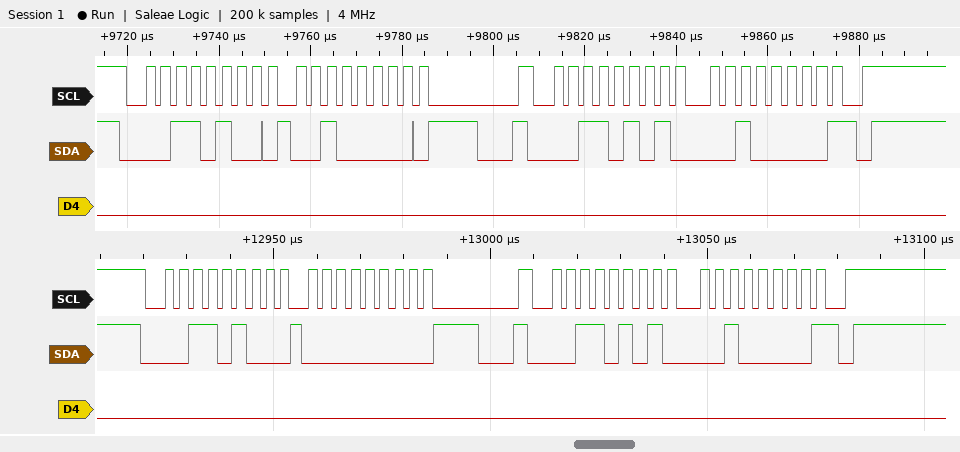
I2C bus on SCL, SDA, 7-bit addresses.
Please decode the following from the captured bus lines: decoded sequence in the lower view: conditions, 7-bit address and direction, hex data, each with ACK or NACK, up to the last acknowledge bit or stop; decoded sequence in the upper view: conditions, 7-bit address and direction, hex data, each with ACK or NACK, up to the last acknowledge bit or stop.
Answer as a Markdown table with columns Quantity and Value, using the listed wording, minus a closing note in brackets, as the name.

| Quantity | Value |
|---|---|
| decoded sequence in the lower view: conditions, 7-bit address and direction, hex data, each with ACK or NACK, up to the last acknowledge bit or stop | start, address 1A write ACK, 00 ACK, repeated start, address 1A read ACK, 20 NACK, stop |
| decoded sequence in the upper view: conditions, 7-bit address and direction, hex data, each with ACK or NACK, up to the last acknowledge bit or stop | start, address 1A write ACK, 20 ACK, repeated start, address 1A read ACK, 20 NACK, stop |
